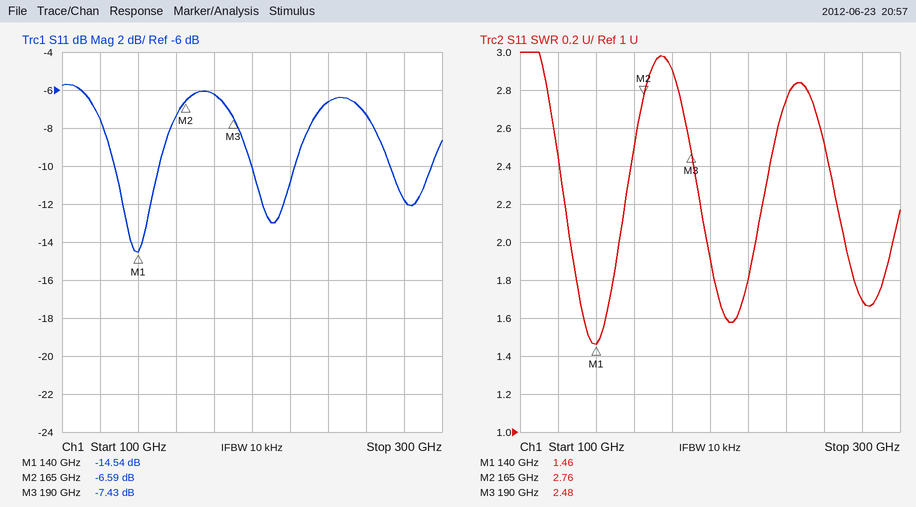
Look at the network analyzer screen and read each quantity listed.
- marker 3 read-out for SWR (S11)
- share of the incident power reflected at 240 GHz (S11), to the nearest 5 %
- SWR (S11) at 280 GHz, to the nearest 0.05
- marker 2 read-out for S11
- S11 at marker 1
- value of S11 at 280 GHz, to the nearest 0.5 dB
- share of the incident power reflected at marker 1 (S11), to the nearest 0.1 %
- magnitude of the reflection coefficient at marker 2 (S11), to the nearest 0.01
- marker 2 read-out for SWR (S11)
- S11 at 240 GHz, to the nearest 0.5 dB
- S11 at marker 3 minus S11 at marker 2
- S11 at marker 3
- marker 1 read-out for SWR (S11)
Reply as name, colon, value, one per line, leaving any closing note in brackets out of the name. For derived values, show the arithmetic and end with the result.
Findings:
marker 3 read-out for SWR: 2.48
share of the incident power reflected at 240 GHz (S11), to the nearest 5 %: 10^(-6.5/10) ≈ 22.4 %, so 20 % to the nearest 5 %
SWR (S11) at 280 GHz, to the nearest 0.05: 1.70
marker 2 read-out for S11: -6.59 dB
S11 at marker 1: -14.54 dB
value of S11 at 280 GHz, to the nearest 0.5 dB: -12.0 dB
share of the incident power reflected at marker 1 (S11), to the nearest 0.1 %: 10^(-14.54/10) ≈ 3.5 %
magnitude of the reflection coefficient at marker 2 (S11), to the nearest 0.01: 10^(-6.59/20) ≈ 0.47
marker 2 read-out for SWR: 2.76
S11 at 240 GHz, to the nearest 0.5 dB: -6.5 dB
S11 at marker 3 minus S11 at marker 2: -7.43 − (-6.59) = -0.84 dB
S11 at marker 3: -7.43 dB
marker 1 read-out for SWR: 1.46
